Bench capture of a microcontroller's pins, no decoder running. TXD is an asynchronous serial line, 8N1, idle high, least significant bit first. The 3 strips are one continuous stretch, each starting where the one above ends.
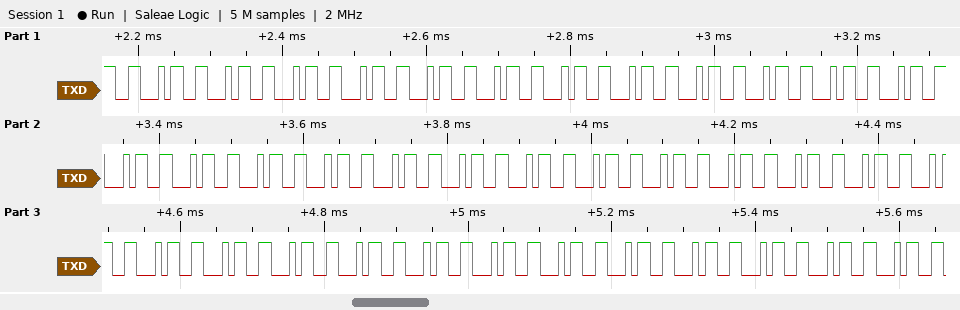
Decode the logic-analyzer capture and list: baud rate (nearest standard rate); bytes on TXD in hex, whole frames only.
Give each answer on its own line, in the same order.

115200 baud
0x46 0x46 0x46 0x46 0x46 0x46 0x46 0x46 0x46 0x46 0x46 0x46 0x46 0x46 0x46 0x46 0x46 0x46 0x46 0x46 0x46 0x46 0x46 0x46 0x46 0x46 0x46 0x46 0x46 0x46 0x46 0x46 0x46 0x46 0x46 0x46 0x46
